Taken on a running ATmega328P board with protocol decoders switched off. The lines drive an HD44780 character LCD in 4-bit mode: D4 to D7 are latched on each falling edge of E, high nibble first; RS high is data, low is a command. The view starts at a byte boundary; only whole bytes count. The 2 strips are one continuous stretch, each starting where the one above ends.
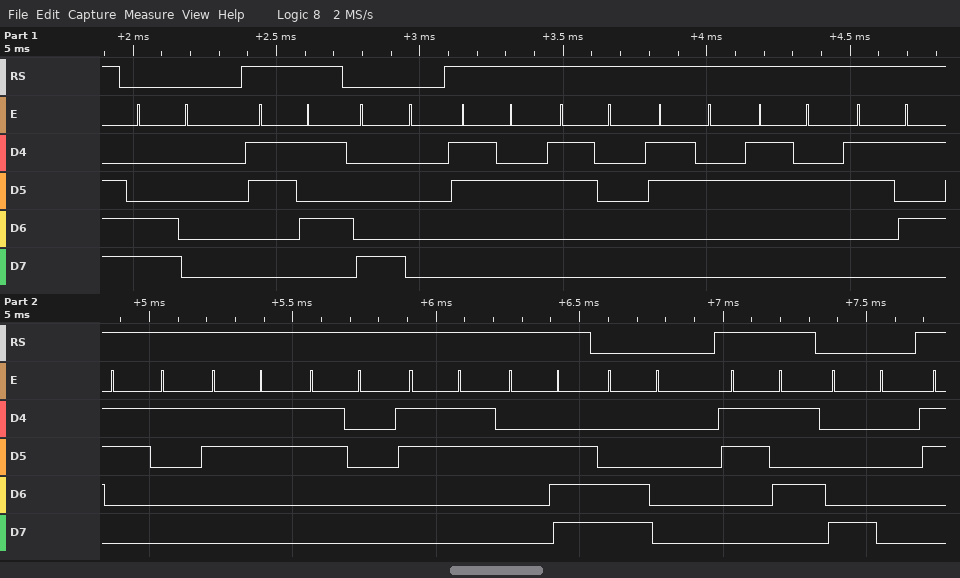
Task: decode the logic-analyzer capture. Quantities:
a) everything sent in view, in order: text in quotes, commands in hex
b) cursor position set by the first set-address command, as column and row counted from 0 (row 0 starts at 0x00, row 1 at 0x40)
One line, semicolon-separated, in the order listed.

0xC0 "5" 0x80 "202251303." 0xC0 "5" 0x80; column 0, row 1
